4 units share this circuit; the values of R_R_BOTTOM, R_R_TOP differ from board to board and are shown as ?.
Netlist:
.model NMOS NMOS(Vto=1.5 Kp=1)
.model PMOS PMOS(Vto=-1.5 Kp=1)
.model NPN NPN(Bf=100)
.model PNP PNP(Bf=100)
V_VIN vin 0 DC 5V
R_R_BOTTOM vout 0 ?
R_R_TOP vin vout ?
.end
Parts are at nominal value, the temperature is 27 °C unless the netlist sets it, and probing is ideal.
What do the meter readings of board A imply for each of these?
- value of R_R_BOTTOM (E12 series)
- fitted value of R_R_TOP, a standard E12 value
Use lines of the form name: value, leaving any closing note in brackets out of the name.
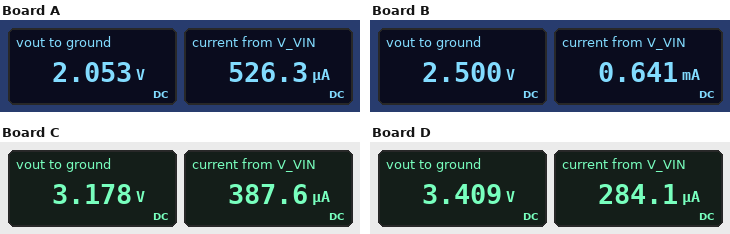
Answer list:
value of R_R_BOTTOM: 3.9 kΩ
fitted value of R_R_TOP, a standard E12 value: 5.6 kΩ
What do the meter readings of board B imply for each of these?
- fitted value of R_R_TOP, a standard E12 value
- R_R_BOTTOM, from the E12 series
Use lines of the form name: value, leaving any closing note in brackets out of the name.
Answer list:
fitted value of R_R_TOP, a standard E12 value: 3.9 kΩ
R_R_BOTTOM, from the E12 series: 3.9 kΩ
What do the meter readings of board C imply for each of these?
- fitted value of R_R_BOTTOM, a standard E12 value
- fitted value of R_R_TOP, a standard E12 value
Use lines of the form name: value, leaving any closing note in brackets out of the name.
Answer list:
fitted value of R_R_BOTTOM, a standard E12 value: 8.2 kΩ
fitted value of R_R_TOP, a standard E12 value: 4.7 kΩ
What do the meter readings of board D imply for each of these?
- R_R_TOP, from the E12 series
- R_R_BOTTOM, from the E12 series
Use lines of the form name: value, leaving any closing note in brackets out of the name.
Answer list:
R_R_TOP, from the E12 series: 5.6 kΩ
R_R_BOTTOM, from the E12 series: 12 kΩ
